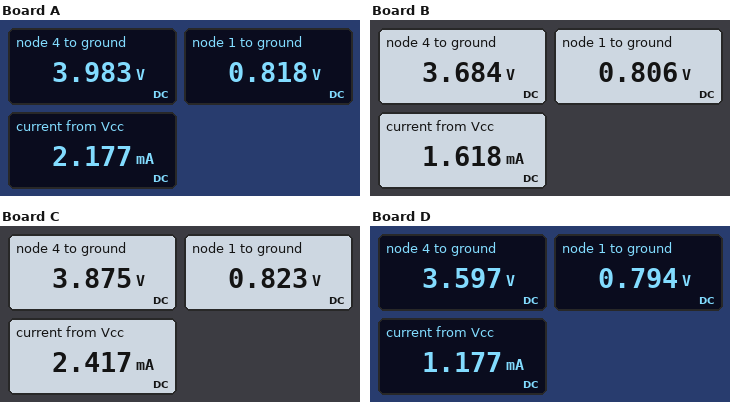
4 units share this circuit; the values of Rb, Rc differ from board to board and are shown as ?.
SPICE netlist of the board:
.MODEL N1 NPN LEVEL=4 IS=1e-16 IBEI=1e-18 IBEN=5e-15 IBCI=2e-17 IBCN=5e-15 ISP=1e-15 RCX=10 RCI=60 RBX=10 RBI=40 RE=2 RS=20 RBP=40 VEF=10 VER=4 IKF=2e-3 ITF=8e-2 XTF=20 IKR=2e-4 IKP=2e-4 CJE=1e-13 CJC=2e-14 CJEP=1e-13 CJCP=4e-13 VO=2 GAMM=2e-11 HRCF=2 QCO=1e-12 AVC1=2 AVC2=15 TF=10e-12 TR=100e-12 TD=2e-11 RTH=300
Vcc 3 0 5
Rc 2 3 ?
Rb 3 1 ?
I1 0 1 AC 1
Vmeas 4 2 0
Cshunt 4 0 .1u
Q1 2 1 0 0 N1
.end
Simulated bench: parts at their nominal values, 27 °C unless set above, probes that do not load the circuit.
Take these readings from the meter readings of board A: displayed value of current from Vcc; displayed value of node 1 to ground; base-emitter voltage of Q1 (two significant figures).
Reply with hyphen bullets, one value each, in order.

- 2.177 mA
- 0.818 V
- 820 mV
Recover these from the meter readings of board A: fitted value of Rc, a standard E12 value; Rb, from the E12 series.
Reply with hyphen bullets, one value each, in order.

- 470 Ω
- 330 kΩ
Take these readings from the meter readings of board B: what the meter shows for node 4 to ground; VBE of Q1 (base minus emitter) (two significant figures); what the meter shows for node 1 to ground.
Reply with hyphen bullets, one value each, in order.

- 3.684 V
- 810 mV
- 0.806 V
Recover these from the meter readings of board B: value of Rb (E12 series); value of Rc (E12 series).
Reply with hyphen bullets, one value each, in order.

- 330 kΩ
- 820 Ω
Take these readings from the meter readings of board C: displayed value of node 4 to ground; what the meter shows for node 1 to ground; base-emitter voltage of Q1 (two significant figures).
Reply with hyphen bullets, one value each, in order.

- 3.875 V
- 0.823 V
- 820 mV
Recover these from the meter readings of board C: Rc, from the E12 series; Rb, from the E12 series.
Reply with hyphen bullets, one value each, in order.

- 470 Ω
- 180 kΩ
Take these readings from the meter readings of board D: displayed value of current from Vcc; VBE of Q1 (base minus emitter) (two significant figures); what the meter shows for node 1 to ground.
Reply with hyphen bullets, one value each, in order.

- 1.177 mA
- 790 mV
- 0.794 V
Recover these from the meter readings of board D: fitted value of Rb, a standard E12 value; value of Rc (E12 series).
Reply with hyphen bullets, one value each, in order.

- 560 kΩ
- 1.2 kΩ
